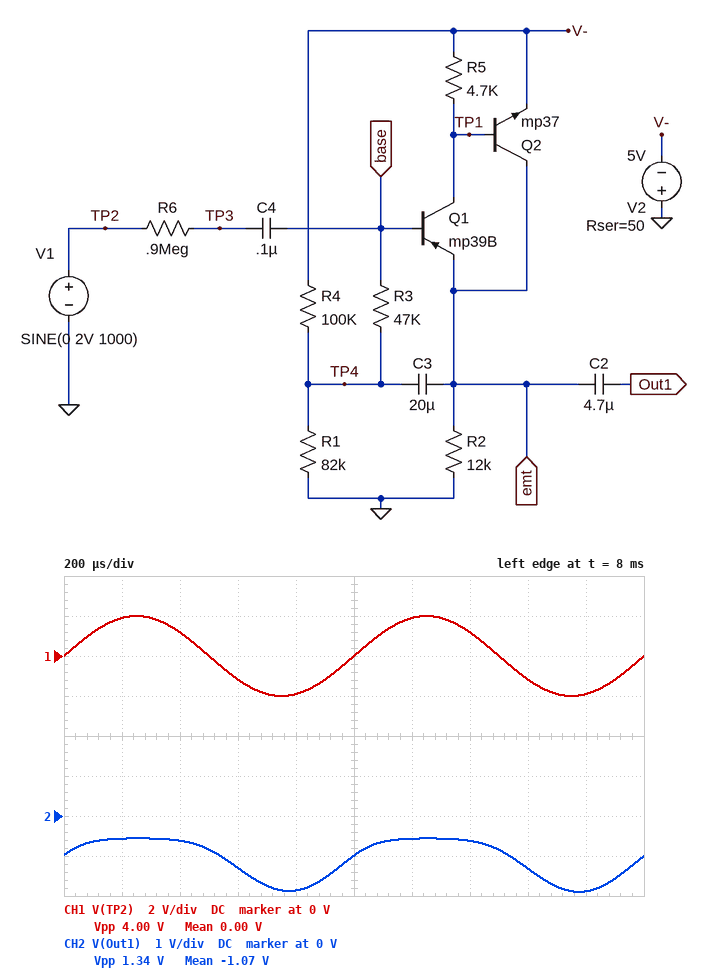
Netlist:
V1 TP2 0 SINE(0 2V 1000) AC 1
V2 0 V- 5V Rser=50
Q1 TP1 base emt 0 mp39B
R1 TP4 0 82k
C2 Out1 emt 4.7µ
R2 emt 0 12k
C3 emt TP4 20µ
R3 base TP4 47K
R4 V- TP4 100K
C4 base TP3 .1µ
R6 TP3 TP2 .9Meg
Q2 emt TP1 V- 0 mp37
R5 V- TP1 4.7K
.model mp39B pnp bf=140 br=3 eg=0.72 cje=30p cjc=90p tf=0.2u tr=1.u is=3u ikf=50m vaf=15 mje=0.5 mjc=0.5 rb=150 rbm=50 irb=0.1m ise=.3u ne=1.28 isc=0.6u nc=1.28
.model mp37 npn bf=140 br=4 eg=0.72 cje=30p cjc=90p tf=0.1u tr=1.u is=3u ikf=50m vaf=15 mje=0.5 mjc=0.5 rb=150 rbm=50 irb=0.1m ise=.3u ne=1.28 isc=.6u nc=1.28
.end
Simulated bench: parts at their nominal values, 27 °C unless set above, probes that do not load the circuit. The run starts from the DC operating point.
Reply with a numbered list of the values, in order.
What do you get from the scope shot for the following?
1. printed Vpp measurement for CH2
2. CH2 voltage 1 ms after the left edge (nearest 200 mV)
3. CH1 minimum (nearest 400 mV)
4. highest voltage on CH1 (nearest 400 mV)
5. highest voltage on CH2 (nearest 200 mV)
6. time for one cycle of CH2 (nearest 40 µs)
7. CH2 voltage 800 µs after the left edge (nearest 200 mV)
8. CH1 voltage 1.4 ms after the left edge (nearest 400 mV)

1. 1.34 V
2. -1.0 V
3. -2.0 V
4. 2.0 V
5. -600 mV
6. 1.00 ms
7. -1.8 V
8. 1.2 V
